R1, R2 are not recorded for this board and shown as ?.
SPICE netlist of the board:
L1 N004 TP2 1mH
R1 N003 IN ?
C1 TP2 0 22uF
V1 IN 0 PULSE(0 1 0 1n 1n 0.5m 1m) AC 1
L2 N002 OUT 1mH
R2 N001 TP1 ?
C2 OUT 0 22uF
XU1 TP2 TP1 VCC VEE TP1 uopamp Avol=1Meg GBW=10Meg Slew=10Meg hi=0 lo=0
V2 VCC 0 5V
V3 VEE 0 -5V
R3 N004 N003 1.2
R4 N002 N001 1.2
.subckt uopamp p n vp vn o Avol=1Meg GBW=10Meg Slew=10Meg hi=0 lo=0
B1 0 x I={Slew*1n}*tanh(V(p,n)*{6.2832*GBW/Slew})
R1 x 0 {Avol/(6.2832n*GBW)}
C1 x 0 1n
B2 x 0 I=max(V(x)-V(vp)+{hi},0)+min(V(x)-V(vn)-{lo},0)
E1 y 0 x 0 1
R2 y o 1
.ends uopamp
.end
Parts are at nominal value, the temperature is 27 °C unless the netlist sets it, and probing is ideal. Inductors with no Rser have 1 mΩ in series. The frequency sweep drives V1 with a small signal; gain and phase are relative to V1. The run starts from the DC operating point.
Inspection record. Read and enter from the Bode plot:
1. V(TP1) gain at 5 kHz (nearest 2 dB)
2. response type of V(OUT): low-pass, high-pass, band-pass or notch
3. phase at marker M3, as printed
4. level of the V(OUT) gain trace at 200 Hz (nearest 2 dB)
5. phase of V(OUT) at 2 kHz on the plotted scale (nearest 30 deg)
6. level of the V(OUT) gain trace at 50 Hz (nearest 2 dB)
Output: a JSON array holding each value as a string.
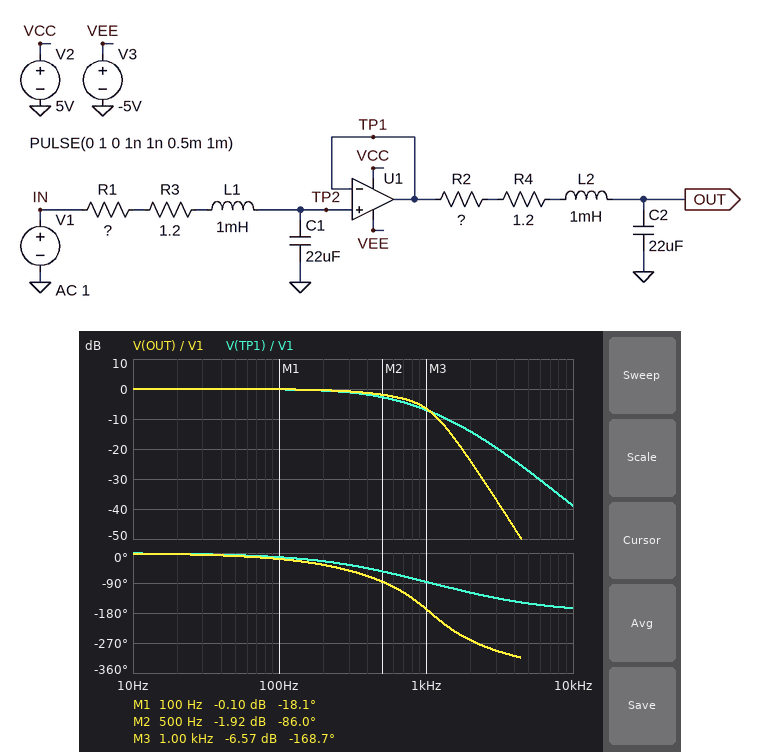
["-28 dB", "low-pass", "-168.7 deg", "0 dB", "-270 deg", "0 dB"]
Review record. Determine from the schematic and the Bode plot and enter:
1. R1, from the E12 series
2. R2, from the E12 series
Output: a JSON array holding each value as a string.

["15 Ω", "5.6 Ω"]
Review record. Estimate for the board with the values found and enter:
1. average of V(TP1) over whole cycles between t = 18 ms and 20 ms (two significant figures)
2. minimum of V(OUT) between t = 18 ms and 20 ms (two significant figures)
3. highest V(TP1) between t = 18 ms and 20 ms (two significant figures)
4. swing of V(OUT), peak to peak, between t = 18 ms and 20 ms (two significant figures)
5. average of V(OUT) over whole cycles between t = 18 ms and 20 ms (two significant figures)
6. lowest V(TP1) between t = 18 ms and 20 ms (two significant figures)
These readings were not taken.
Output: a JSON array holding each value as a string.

["500 mV", "200 mV", "810 mV", "600 mV", "500 mV", "190 mV"]
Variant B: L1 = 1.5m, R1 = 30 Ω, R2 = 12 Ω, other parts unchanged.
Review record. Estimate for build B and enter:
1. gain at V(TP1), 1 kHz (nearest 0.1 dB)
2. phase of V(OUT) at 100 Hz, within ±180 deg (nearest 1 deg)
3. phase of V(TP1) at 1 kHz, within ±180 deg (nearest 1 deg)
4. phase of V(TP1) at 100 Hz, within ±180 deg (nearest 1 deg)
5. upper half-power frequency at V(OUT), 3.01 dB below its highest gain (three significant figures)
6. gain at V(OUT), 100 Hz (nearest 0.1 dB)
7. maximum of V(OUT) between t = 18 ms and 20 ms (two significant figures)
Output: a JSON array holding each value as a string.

["-12.7 dB", "-34 deg", "-94 deg", "-24 deg", "229 Hz", "-0.7 dB", "580 mV"]
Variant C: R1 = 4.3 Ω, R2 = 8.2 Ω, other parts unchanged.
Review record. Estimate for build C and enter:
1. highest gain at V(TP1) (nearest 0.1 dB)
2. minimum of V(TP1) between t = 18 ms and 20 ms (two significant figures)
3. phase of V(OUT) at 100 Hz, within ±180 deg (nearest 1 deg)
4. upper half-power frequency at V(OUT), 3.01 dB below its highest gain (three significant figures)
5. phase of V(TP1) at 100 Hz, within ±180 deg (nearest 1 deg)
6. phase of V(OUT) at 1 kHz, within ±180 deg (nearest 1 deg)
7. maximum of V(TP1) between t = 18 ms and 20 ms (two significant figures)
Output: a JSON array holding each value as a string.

["2.6 dB", "-320 mV", "-12 deg", "1.10 kHz", "-4 deg", "-164 deg", "1.3 V"]
